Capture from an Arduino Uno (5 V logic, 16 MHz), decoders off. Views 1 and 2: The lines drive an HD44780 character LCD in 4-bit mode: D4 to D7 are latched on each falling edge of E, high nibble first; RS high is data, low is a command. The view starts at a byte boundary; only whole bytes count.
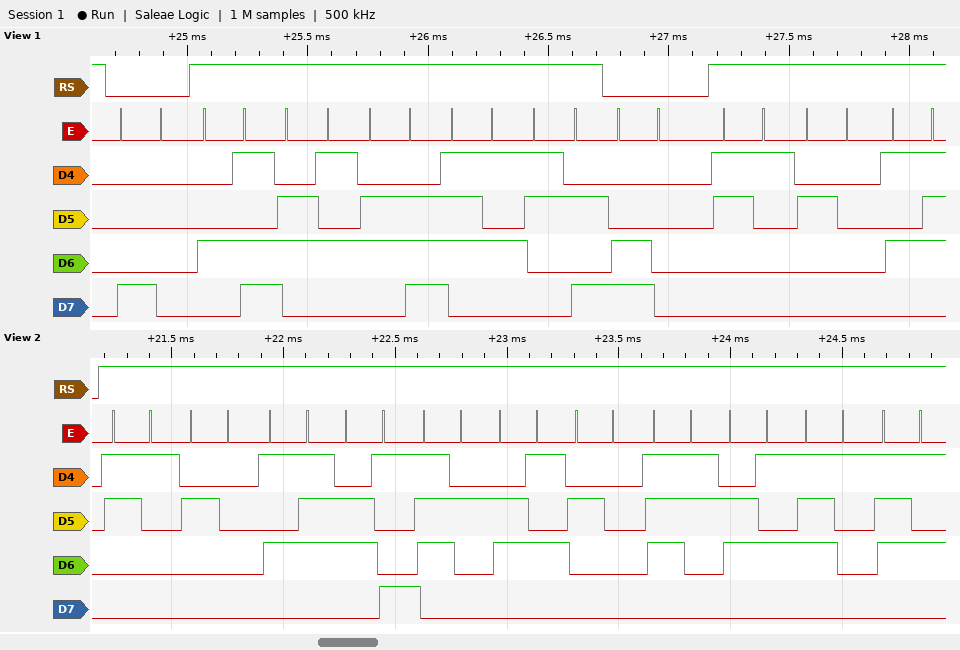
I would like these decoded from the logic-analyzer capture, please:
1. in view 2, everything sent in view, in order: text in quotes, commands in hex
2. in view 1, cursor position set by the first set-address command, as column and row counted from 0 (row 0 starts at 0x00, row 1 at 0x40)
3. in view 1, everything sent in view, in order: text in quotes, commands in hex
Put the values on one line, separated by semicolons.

"1 Wire sequ"; column 0, row 0; 0x80 "Menu:" 0xC0 "1 W"
